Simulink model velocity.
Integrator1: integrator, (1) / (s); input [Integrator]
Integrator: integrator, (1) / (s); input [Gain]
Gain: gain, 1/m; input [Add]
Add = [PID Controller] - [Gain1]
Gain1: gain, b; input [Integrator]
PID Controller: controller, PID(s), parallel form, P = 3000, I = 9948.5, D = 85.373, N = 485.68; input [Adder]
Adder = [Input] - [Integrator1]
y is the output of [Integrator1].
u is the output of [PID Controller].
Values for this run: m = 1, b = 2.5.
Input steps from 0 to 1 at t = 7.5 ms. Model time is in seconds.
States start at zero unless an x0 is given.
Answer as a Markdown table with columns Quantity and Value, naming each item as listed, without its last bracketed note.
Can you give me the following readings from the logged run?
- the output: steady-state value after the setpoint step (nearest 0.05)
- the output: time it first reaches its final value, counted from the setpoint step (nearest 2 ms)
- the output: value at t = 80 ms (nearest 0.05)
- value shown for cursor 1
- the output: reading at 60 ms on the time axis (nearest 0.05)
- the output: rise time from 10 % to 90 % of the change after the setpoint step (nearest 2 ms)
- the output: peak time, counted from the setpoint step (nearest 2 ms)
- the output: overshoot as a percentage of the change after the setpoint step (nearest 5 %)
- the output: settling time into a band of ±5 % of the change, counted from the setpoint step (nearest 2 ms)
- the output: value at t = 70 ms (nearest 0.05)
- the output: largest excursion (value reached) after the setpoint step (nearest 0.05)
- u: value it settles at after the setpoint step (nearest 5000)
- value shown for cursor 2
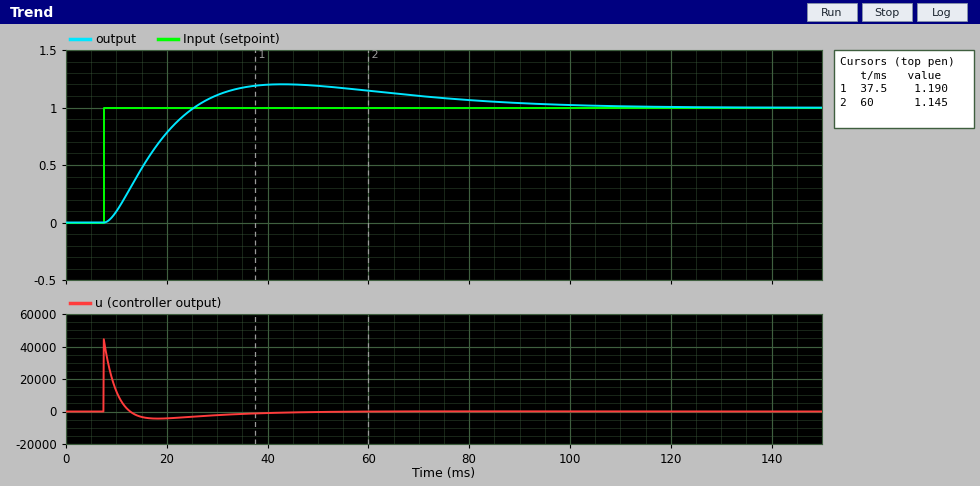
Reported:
| Quantity | Value |
|---|---|
| the output: steady-state value after the setpoint step | 1.00 |
| the output: time it first reaches its final value, counted from the setpoint step | 18 ms |
| the output: value at t = 80 ms | 1.05 |
| value shown for cursor 1 | 1.190 |
| the output: reading at 60 ms on the time axis | 1.15 |
| the output: rise time from 10 % to 90 % of the change after the setpoint step | 12 ms |
| the output: peak time, counted from the setpoint step | 36 ms |
| the output: overshoot as a percentage of the change after the setpoint step | 20 % |
| the output: settling time into a band of ±5 % of the change, counted from the setpoint step | 78 ms |
| the output: value at t = 70 ms | 1.10 |
| the output: largest excursion (value reached) after the setpoint step | 1.20 |
| u: value it settles at after the setpoint step | 0 |
| value shown for cursor 2 | 1.145 |
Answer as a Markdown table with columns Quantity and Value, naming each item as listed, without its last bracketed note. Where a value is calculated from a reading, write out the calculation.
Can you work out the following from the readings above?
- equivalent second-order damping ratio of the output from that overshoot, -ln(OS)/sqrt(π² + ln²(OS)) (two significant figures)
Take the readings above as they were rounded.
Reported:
| Quantity | Value |
|---|---|
| equivalent second-order damping ratio of the output from that overshoot, -ln(OS)/sqrt(π² + ln²(OS)) | ln(0.2) = -1.609; 1.609 / sqrt(9.870 + 2.590) = 0.46 |
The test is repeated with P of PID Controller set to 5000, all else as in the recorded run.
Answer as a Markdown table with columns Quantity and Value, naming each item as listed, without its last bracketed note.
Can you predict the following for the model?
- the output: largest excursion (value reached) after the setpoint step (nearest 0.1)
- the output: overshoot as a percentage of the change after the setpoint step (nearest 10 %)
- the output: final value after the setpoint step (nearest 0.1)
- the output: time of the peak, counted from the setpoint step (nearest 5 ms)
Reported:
| Quantity | Value |
|---|---|
| the output: largest excursion (value reached) after the setpoint step | 1.3 |
| the output: overshoot as a percentage of the change after the setpoint step | 30 % |
| the output: final value after the setpoint step | 1.0 |
| the output: time of the peak, counted from the setpoint step | 30 ms |
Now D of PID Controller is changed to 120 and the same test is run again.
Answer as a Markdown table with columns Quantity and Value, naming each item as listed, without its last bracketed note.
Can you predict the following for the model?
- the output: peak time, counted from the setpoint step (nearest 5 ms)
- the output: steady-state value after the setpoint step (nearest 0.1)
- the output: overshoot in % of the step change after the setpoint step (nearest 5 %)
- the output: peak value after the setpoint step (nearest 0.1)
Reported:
| Quantity | Value |
|---|---|
| the output: peak time, counted from the setpoint step | 30 ms |
| the output: steady-state value after the setpoint step | 1.0 |
| the output: overshoot in % of the step change after the setpoint step | 15 % |
| the output: peak value after the setpoint step | 1.1 |
